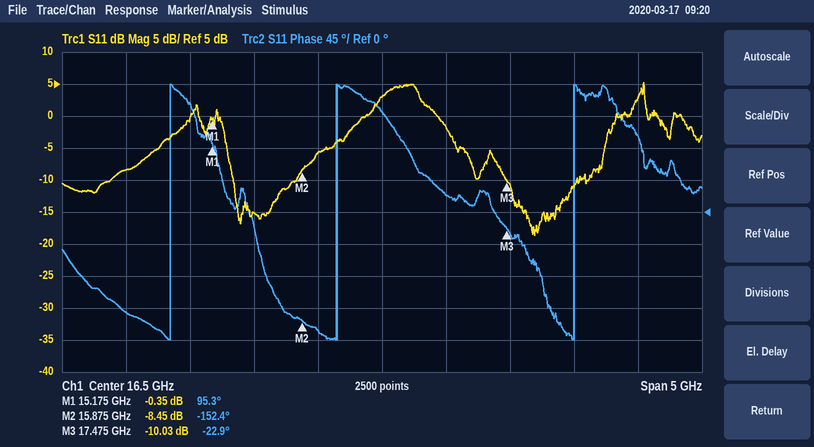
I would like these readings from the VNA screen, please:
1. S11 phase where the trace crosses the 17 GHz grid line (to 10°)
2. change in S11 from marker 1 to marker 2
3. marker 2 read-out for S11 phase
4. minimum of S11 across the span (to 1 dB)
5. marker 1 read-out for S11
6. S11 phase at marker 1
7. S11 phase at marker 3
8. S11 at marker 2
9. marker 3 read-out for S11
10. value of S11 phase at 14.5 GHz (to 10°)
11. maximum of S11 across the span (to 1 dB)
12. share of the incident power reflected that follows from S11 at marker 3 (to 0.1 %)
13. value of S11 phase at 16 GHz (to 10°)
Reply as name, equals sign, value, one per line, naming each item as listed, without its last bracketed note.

S11 phase where the trace crosses the 17 GHz grid line = 20°
change in S11 from marker 1 to marker 2 = -8.10 dB
marker 2 read-out for S11 phase = -152.4°
minimum of S11 across the span = -19 dB
marker 1 read-out for S11 = -0.35 dB
S11 phase at marker 1 = 95.3°
S11 phase at marker 3 = -22.9°
S11 at marker 2 = -8.45 dB
marker 3 read-out for S11 = -10.03 dB
value of S11 phase at 14.5 GHz = -140°
maximum of S11 across the span = 5 dB
share of the incident power reflected that follows from S11 at marker 3 = 9.9 %
value of S11 phase at 16 GHz = -170°
